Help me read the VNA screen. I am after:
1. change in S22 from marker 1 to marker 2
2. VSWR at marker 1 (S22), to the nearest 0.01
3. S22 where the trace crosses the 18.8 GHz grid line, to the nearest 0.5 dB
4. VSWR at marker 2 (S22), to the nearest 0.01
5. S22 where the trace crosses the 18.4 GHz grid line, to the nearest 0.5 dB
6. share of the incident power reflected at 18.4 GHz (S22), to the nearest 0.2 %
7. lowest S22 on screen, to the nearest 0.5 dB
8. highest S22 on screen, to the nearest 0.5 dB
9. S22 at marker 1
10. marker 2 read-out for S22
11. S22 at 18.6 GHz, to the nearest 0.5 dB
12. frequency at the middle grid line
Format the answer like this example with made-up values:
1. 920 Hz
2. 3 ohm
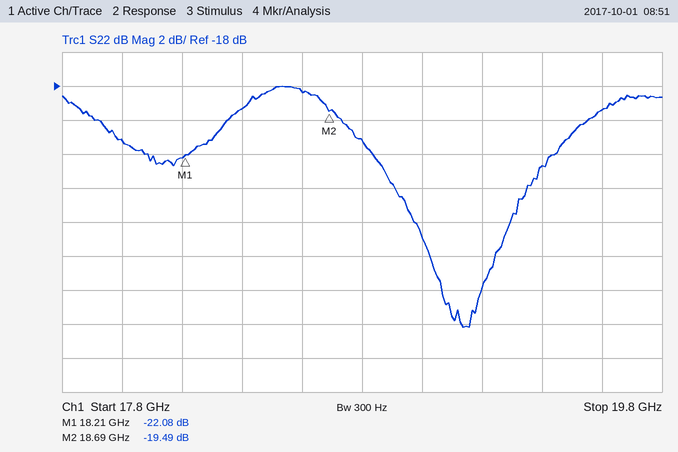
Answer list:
1. 2.59 dB
2. 1.17
3. -21.0 dB
4. 1.24
5. -19.5 dB
6. 1.2 %
7. -32.0 dB
8. -18.0 dB
9. -22.08 dB
10. -19.49 dB
11. -18.5 dB
12. 18.8 GHz
